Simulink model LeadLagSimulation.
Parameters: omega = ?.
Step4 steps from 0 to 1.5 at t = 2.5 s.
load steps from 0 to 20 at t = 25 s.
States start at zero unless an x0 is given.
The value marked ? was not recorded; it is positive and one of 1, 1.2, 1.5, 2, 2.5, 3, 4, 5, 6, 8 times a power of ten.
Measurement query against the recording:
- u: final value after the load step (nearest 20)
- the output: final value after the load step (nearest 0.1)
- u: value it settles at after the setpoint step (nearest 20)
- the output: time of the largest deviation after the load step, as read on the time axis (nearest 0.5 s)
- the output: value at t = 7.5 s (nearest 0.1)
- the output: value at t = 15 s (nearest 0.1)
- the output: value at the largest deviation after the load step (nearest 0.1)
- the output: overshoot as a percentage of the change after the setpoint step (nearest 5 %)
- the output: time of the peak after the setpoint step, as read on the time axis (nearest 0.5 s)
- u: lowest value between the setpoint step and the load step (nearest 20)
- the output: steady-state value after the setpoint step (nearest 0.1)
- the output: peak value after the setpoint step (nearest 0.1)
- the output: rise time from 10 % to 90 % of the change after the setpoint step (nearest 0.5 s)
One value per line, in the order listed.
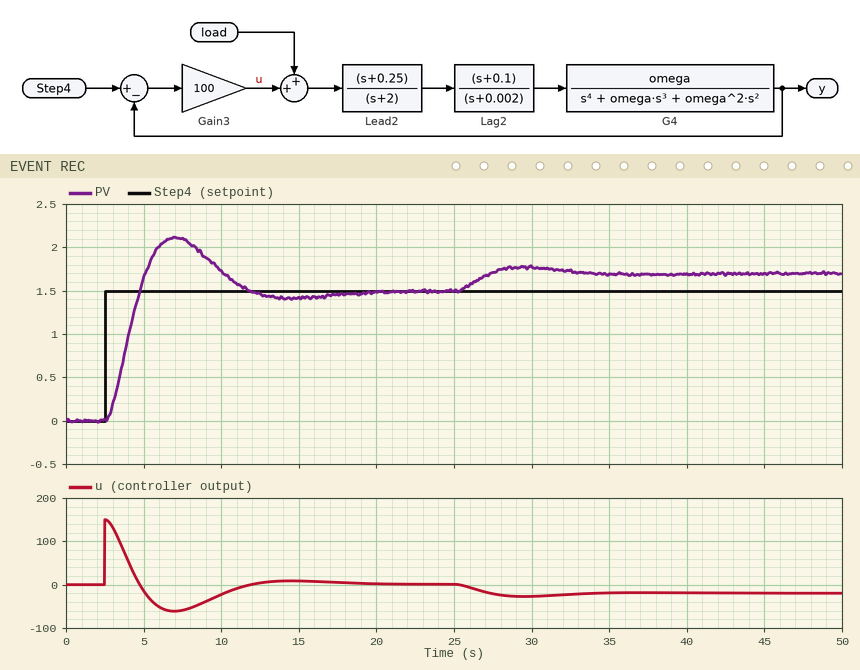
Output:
-20
1.7
0
29.5 s
2.1
1.4
1.8
40 %
7.0 s
-60
1.5
2.1
1.5 s
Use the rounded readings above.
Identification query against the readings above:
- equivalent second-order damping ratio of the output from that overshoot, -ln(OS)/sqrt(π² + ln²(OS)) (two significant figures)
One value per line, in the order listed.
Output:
0.28
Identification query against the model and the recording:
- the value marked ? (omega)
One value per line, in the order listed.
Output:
80
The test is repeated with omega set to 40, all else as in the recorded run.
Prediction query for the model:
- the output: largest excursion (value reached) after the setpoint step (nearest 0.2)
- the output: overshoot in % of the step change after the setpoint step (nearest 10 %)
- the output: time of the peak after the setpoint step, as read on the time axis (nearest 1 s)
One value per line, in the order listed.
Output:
2.0
40 %
5 s
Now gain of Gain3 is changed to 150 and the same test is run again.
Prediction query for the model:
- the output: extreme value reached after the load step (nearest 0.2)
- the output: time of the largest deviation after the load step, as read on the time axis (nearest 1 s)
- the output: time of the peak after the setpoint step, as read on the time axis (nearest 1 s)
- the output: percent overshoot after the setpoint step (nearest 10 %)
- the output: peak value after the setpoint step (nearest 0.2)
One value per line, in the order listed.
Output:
1.6
28 s
6 s
40 %
2.0
